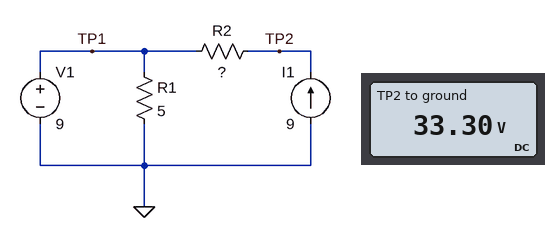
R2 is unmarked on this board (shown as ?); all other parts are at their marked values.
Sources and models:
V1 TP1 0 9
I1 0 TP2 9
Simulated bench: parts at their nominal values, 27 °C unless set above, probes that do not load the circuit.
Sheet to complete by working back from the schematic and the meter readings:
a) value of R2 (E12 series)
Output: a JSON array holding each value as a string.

["2.7 Ω"]
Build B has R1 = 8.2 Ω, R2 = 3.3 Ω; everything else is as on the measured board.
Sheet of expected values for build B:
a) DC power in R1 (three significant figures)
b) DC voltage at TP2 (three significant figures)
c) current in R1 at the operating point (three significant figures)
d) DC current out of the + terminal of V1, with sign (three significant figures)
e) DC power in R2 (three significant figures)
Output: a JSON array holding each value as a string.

["9.88 W", "38.7 V", "1.10 A", "-7.90 A", "267 W"]
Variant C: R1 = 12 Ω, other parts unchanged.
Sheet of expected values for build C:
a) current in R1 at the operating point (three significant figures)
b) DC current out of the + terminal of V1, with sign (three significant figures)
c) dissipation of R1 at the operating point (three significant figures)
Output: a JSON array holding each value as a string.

["750 mA", "-8.25 A", "6.75 W"]
